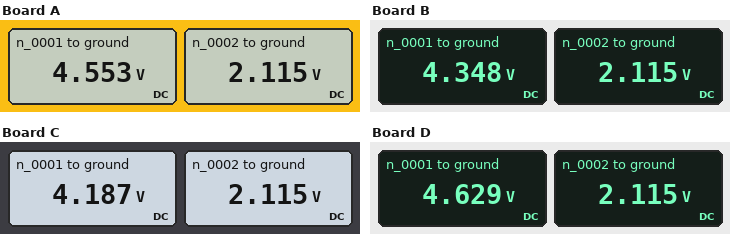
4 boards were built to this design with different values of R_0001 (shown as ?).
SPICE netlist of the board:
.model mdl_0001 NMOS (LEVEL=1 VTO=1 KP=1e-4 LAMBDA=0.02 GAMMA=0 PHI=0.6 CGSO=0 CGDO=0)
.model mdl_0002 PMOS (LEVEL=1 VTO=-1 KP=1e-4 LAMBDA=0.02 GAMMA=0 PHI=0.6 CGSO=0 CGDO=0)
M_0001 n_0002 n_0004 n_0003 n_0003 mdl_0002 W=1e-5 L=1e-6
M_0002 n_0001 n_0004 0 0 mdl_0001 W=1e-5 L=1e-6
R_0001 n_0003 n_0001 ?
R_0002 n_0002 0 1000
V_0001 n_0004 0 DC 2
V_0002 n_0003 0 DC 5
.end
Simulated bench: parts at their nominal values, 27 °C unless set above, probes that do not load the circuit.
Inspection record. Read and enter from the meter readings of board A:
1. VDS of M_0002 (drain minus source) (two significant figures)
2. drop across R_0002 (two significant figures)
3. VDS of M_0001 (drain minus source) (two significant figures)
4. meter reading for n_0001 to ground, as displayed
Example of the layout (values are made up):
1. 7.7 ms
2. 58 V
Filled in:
1. 4.6 V
2. 2.1 V
3. -2.9 V
4. 4.553 V
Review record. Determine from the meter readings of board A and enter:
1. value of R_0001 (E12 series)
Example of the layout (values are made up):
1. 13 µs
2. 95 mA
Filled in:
1. 820 Ω
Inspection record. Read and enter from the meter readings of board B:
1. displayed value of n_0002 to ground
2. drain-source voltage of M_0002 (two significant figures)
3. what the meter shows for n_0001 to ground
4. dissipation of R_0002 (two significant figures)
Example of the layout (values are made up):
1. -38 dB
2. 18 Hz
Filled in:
1. 2.115 V
2. 4.3 V
3. 4.348 V
4. 4.5 mW
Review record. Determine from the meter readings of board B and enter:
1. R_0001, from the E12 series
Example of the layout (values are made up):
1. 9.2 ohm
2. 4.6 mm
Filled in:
1. 1.2 kΩ
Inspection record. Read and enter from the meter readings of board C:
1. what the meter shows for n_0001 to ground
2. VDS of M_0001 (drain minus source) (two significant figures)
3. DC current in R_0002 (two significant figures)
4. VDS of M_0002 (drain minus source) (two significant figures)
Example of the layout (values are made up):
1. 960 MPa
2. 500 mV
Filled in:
1. 4.187 V
2. -2.9 V
3. 2.1 mA
4. 4.2 V
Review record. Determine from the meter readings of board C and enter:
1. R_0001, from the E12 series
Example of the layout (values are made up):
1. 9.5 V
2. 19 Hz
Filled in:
1. 1.5 kΩ
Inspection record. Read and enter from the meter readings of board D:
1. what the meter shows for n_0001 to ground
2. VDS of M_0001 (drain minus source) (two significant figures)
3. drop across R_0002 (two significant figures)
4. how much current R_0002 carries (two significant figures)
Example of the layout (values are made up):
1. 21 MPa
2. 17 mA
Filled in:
1. 4.629 V
2. -2.9 V
3. 2.1 V
4. 2.1 mA
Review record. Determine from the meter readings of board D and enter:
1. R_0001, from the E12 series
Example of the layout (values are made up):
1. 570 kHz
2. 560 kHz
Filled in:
1. 680 Ω
